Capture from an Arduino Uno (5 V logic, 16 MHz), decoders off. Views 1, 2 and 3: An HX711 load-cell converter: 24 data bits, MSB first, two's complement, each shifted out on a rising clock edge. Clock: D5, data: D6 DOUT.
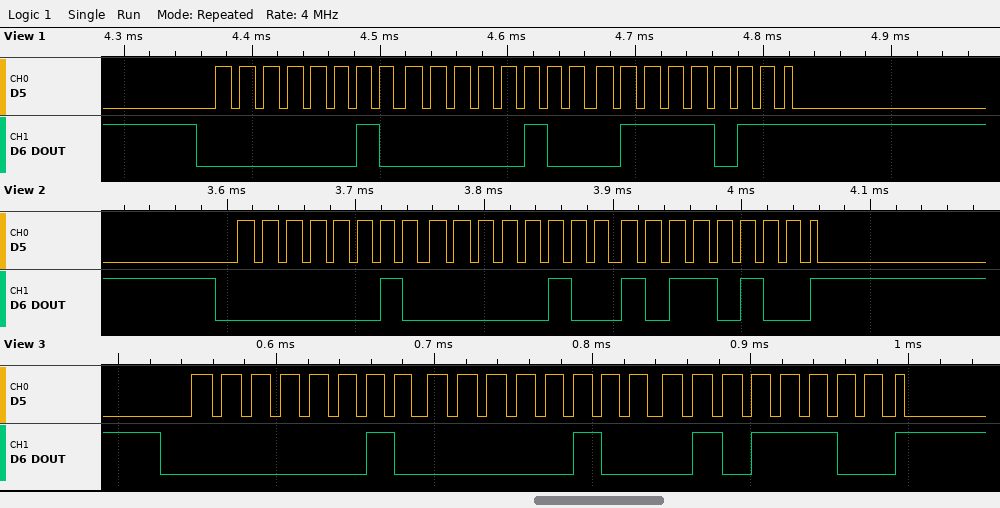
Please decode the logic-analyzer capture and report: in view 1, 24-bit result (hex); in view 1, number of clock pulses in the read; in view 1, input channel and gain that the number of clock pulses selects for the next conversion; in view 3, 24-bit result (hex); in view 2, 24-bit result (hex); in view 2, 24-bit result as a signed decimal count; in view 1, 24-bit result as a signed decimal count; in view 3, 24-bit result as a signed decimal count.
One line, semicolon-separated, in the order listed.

0x02047B; 25; channel A, gain 128; 0x02045C; 0x0204B4; 132276; 132219; 132188
